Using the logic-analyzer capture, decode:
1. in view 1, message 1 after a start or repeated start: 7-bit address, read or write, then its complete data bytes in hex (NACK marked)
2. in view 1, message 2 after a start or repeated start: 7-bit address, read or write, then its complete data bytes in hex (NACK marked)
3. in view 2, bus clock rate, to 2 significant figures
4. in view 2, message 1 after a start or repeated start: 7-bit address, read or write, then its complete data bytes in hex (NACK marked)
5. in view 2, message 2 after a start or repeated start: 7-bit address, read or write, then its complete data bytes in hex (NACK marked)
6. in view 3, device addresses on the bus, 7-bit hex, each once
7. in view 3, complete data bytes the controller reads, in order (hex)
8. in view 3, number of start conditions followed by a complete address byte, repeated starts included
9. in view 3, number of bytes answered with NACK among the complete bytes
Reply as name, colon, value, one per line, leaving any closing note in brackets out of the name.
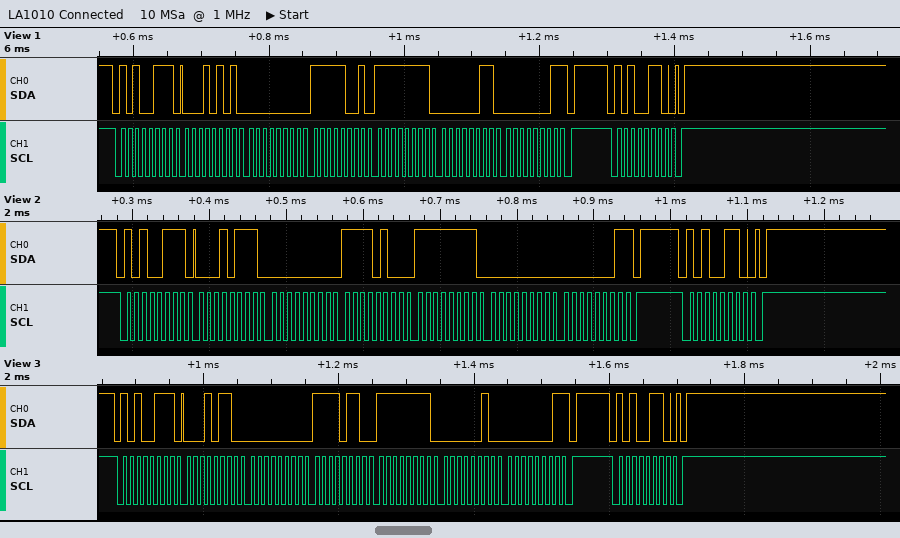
in view 1, message 1 after a start or repeated start: 7-bit address, read or write, then its complete data bytes in hex: 0x53 read: 15 00 F9 FF 03 01 NACK
in view 1, message 2 after a start or repeated start: 7-bit address, read or write, then its complete data bytes in hex: 0x53 write
in view 2, bus clock rate, to 2 significant figures: 100 kHz
in view 2, message 1 after a start or repeated start: 7-bit address, read or write, then its complete data bytes in hex: 0x53 read: 17 00 F4 FF 00 01 NACK
in view 2, message 2 after a start or repeated start: 7-bit address, read or write, then its complete data bytes in hex: 0x53 write
in view 3, device addresses on the bus, 7-bit hex, each once: 0x53
in view 3, complete data bytes the controller reads, in order: 16 00 F6 FF 02 01
in view 3, number of start conditions followed by a complete address byte, repeated starts included: 2
in view 3, number of bytes answered with NACK among the complete bytes: 1
